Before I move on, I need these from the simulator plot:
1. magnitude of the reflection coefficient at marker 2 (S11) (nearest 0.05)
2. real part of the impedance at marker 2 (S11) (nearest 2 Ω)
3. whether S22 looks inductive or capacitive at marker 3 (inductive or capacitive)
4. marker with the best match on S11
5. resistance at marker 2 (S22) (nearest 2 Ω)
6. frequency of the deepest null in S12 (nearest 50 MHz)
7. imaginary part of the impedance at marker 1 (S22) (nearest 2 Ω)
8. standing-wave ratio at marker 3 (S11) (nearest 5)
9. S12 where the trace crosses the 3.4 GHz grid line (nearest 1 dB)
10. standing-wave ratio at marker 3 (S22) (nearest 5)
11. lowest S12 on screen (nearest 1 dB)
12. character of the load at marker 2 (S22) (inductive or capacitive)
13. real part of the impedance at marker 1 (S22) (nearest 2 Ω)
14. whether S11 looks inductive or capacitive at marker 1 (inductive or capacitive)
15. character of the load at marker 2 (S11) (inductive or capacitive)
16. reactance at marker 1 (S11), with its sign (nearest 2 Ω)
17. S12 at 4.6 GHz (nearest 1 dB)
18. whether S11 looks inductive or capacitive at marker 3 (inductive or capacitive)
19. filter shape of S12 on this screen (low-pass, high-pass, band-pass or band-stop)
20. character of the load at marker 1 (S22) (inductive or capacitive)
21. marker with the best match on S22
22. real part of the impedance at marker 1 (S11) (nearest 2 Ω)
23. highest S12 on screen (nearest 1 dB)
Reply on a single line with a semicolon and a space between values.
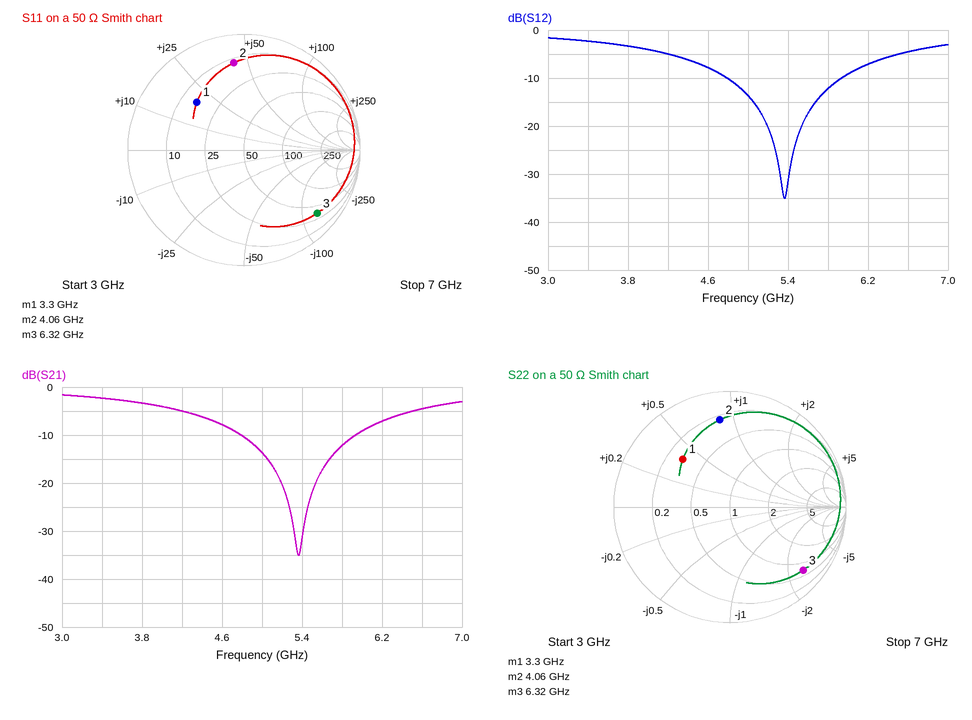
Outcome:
0.75; 12 Ω; capacitive; marker 1; 12 Ω; 5.35 GHz; +20 Ω; 10; -2 dB; 10; -35 dB; inductive; 16 Ω; inductive; inductive; +20 Ω; -8 dB; capacitive; band-stop; inductive; marker 1; 16 Ω; -2 dB
